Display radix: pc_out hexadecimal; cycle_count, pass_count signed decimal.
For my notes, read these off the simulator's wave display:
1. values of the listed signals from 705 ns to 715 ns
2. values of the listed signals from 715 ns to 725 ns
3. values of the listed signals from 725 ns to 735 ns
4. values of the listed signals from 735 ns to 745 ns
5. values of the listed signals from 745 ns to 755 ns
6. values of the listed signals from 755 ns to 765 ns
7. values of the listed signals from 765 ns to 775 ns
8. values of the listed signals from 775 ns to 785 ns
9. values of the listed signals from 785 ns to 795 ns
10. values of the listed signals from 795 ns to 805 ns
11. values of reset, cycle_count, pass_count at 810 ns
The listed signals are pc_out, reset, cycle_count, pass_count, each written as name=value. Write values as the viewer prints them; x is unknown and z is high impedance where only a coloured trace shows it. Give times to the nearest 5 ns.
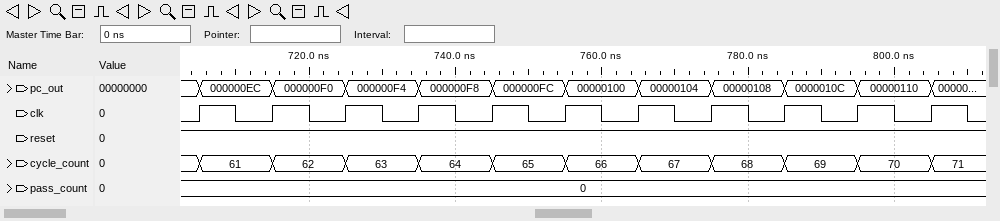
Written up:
pc_out=000000EC, reset=1, cycle_count=61, pass_count=0
pc_out=000000F0, reset=1, cycle_count=62, pass_count=0
pc_out=000000F4, reset=1, cycle_count=63, pass_count=0
pc_out=000000F8, reset=1, cycle_count=64, pass_count=0
pc_out=000000FC, reset=1, cycle_count=65, pass_count=0
pc_out=00000100, reset=1, cycle_count=66, pass_count=0
pc_out=00000104, reset=1, cycle_count=67, pass_count=0
pc_out=00000108, reset=1, cycle_count=68, pass_count=0
pc_out=0000010C, reset=1, cycle_count=69, pass_count=0
pc_out=00000110, reset=1, cycle_count=70, pass_count=0
reset=1, cycle_count=71, pass_count=0
